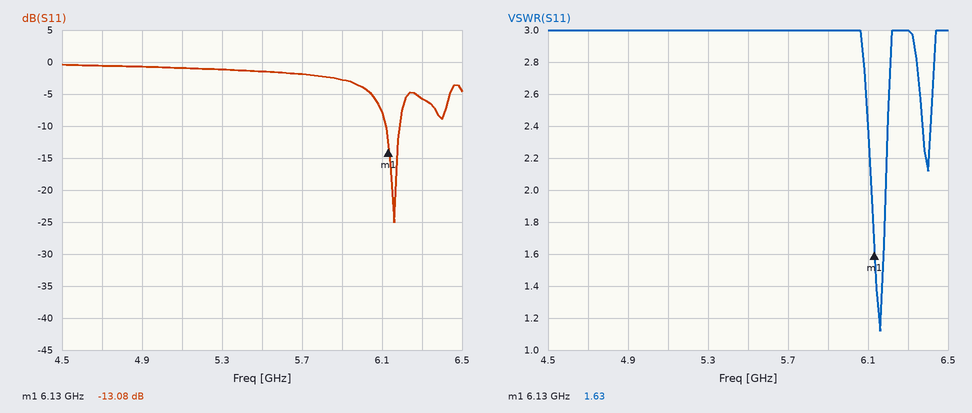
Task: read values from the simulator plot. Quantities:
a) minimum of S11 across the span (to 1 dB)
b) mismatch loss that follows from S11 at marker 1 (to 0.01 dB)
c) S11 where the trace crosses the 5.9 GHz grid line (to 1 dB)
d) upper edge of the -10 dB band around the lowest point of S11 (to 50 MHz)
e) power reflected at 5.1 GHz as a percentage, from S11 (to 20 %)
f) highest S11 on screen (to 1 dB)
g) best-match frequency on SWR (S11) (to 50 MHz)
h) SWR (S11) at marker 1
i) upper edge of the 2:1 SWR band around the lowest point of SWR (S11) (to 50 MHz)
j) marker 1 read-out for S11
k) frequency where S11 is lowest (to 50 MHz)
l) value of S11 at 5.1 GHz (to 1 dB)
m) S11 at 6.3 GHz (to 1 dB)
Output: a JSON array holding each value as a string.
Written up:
["-25 dB", "0.22 dB", "-3 dB", "6.20 GHz", "80 %", "0 dB", "6.15 GHz", "1.63", "6.20 GHz", "-13.08 dB", "6.15 GHz", "-1 dB", "-6 dB"]
